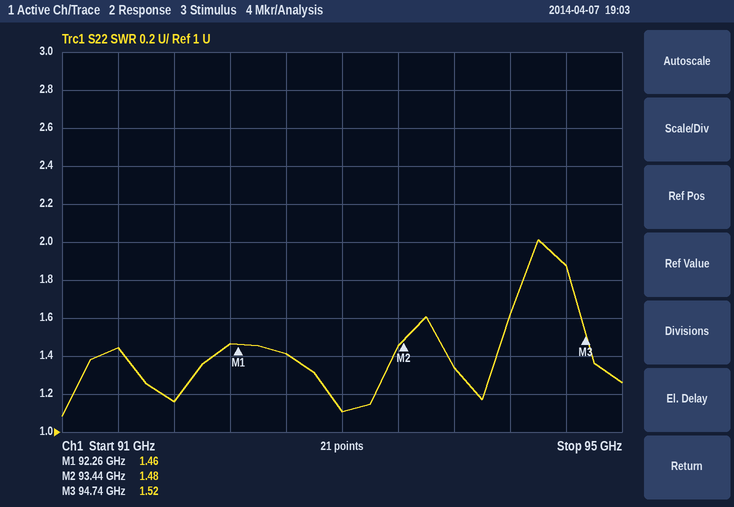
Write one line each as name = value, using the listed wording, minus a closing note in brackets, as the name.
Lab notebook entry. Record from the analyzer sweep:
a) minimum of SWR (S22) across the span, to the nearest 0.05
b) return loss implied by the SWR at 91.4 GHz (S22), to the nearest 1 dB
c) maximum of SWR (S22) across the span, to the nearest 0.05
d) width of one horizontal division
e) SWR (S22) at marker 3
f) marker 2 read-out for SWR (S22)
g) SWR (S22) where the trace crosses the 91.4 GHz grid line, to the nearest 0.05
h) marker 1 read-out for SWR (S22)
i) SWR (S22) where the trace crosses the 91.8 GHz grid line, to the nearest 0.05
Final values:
minimum of SWR (S22) across the span, to the nearest 0.05 = 1.10
return loss implied by the SWR at 91.4 GHz (S22), to the nearest 1 dB = 15 dB
maximum of SWR (S22) across the span, to the nearest 0.05 = 2.00
width of one horizontal division = 400 MHz
SWR (S22) at marker 3 = 1.52
marker 2 read-out for SWR = 1.48
SWR (S22) where the trace crosses the 91.4 GHz grid line, to the nearest 0.05 = 1.45
marker 1 read-out for SWR = 1.46
SWR (S22) where the trace crosses the 91.8 GHz grid line, to the nearest 0.05 = 1.15
